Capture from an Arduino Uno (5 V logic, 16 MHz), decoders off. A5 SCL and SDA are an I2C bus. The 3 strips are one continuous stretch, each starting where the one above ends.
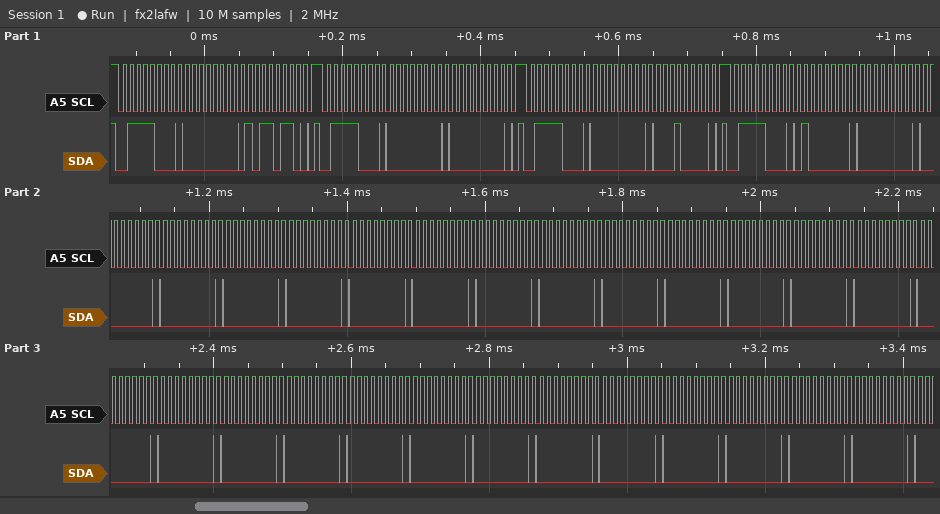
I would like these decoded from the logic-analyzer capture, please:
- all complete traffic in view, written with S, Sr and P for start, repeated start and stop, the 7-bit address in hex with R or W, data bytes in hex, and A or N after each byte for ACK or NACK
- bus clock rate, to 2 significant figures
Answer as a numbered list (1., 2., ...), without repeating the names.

1. S 3CW A 00 A B6 A P S 3CW A 00 A 00 A P S 3CW A 00 A 10 A P S 3CW A 40 A 00 A 00 A 00 A 00 A 00 A 00 A 00 A 00 A 00 A 00 A 00 A 00 A 00 A 00 A 00 A 00 A 00 A 00 A 00 A 00 A 00 A 00 A 00 A 00 A 00 A 00 A 00 A
2. 100 kHz
